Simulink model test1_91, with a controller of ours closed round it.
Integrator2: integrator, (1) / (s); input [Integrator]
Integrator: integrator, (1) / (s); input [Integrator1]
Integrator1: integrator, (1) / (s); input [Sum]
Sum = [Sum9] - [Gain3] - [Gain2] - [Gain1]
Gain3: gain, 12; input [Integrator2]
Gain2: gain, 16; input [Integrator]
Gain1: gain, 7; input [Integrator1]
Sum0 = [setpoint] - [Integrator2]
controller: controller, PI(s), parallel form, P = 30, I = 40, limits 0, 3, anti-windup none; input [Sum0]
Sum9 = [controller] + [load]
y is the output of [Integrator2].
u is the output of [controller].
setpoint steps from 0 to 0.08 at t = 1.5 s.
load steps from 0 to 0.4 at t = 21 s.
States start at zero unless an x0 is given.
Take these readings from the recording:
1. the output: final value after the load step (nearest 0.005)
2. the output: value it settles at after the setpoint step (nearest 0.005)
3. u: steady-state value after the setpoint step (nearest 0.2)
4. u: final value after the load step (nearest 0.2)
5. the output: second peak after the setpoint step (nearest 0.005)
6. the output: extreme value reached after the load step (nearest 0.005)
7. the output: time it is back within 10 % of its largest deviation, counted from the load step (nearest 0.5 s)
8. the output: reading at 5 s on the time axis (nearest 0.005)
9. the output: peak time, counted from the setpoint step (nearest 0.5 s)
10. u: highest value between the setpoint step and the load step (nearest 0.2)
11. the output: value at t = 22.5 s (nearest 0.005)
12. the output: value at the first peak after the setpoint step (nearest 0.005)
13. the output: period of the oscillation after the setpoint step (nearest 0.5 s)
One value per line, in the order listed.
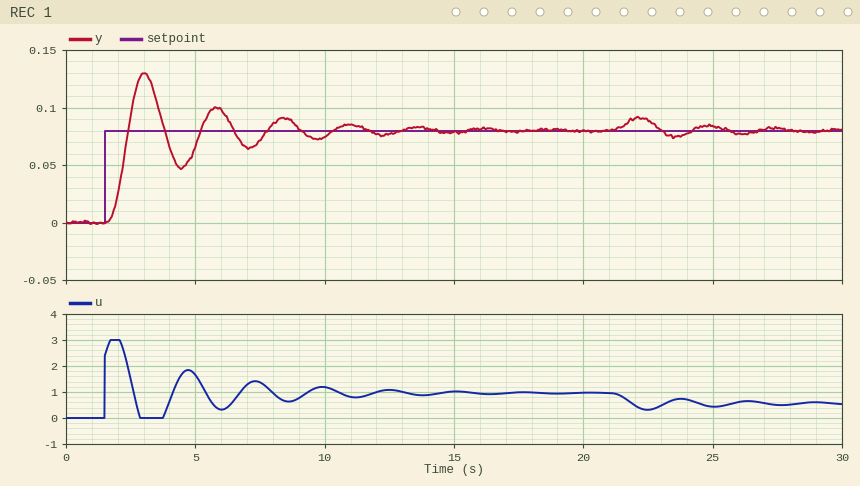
0.080
0.080
1.0
0.6
0.100
0.090
8.0 s
0.065
1.5 s
3.0
0.090
0.130
3.0 s
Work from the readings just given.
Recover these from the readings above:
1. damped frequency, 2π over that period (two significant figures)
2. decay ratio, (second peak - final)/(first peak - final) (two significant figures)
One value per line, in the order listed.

2.1 rad/s
0.40
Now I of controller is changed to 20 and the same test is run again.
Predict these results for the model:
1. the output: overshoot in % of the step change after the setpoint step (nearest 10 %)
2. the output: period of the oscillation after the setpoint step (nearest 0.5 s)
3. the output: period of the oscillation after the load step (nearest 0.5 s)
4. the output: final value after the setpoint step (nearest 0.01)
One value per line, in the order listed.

30 %
2.5 s
2.5 s
0.08
